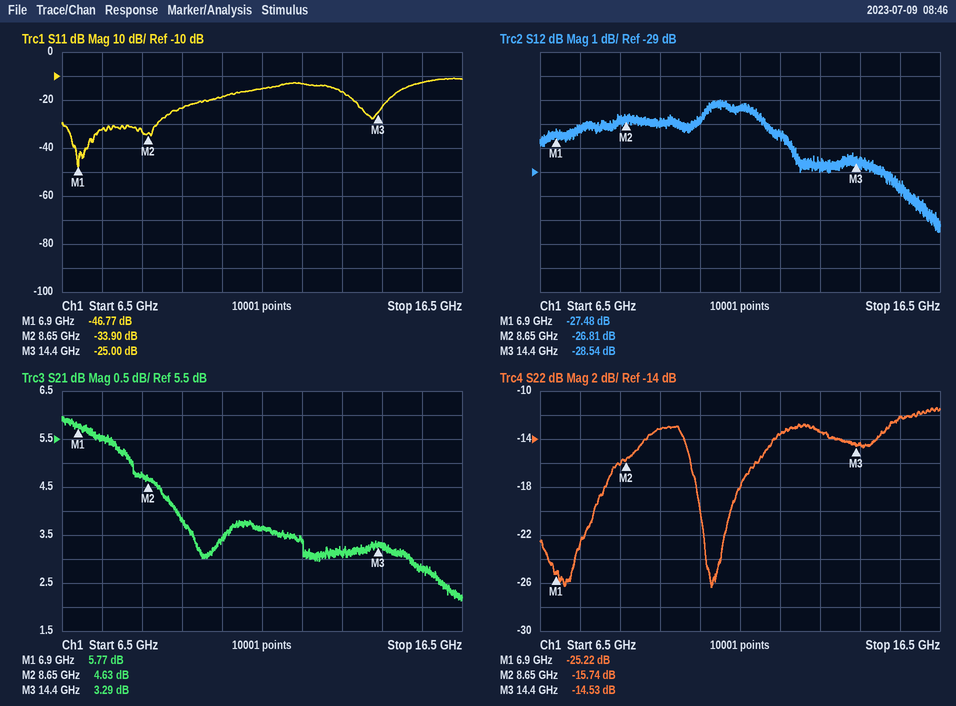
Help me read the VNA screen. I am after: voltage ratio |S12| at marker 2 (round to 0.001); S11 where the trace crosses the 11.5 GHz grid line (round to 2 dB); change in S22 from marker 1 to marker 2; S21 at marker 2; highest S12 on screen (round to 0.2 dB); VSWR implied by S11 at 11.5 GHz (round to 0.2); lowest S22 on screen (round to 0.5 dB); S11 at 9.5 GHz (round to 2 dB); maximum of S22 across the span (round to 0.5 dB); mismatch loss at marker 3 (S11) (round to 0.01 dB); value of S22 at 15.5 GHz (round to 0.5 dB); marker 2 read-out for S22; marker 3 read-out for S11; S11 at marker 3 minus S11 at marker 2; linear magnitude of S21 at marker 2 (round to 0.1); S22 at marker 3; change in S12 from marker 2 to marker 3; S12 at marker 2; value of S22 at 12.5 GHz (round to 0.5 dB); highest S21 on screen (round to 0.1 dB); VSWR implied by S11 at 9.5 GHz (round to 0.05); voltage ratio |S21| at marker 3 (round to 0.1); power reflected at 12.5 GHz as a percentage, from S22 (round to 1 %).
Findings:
0.046
-16 dB
9.48 dB
4.63 dB
-26.0 dB
1.4
-26.5 dB
-24 dB
-11.5 dB
0.01 dB
-12.0 dB
-15.74 dB
-25.00 dB
8.90 dB
1.7
-14.53 dB
-1.73 dB
-26.81 dB
-13.5 dB
6.0 dB
1.15
1.5
4 %
